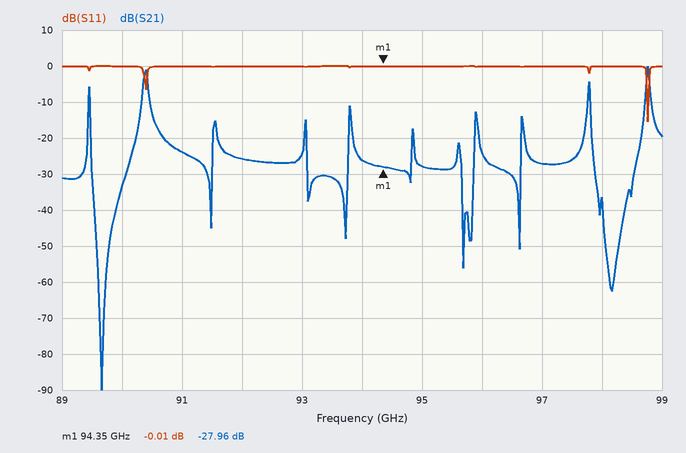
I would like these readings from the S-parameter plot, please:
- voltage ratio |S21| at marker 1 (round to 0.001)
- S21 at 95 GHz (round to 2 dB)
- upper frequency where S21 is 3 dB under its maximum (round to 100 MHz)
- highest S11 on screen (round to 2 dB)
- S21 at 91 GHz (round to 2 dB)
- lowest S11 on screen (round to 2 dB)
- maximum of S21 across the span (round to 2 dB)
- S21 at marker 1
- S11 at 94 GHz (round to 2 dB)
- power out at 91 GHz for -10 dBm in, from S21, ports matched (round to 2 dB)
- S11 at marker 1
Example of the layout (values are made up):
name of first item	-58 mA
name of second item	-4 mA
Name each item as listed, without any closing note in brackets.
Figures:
voltage ratio |S21| at marker 1	0.040
S21 at 95 GHz	-28 dB
upper frequency where S21 is 3 dB under its maximum	98.8 GHz
highest S11 on screen	0 dB
S21 at 91 GHz	-24 dB
lowest S11 on screen	-16 dB
maximum of S21 across the span	0 dB
S21 at marker 1	-27.96 dB
S11 at 94 GHz	0 dB
power out at 91 GHz for -10 dBm in, from S21, ports matched	-34 dBm
S11 at marker 1	-0.01 dB
